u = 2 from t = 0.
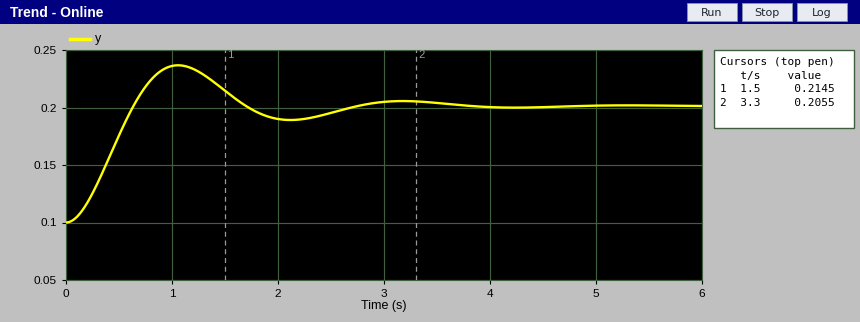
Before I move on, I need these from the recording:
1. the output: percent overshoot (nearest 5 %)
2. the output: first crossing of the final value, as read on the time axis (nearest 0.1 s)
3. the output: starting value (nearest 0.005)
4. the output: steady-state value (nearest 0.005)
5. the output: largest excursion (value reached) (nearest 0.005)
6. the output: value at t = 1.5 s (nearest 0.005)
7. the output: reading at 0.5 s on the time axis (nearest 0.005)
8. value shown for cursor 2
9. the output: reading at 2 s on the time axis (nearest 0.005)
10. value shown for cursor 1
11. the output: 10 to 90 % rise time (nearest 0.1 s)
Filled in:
35 %
0.6 s
0.100
0.200
0.235
0.215
0.175
0.2055
0.190
0.2145
0.4 s
